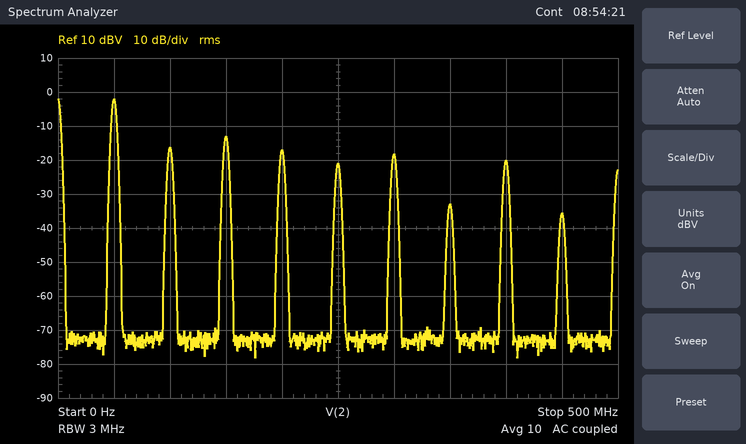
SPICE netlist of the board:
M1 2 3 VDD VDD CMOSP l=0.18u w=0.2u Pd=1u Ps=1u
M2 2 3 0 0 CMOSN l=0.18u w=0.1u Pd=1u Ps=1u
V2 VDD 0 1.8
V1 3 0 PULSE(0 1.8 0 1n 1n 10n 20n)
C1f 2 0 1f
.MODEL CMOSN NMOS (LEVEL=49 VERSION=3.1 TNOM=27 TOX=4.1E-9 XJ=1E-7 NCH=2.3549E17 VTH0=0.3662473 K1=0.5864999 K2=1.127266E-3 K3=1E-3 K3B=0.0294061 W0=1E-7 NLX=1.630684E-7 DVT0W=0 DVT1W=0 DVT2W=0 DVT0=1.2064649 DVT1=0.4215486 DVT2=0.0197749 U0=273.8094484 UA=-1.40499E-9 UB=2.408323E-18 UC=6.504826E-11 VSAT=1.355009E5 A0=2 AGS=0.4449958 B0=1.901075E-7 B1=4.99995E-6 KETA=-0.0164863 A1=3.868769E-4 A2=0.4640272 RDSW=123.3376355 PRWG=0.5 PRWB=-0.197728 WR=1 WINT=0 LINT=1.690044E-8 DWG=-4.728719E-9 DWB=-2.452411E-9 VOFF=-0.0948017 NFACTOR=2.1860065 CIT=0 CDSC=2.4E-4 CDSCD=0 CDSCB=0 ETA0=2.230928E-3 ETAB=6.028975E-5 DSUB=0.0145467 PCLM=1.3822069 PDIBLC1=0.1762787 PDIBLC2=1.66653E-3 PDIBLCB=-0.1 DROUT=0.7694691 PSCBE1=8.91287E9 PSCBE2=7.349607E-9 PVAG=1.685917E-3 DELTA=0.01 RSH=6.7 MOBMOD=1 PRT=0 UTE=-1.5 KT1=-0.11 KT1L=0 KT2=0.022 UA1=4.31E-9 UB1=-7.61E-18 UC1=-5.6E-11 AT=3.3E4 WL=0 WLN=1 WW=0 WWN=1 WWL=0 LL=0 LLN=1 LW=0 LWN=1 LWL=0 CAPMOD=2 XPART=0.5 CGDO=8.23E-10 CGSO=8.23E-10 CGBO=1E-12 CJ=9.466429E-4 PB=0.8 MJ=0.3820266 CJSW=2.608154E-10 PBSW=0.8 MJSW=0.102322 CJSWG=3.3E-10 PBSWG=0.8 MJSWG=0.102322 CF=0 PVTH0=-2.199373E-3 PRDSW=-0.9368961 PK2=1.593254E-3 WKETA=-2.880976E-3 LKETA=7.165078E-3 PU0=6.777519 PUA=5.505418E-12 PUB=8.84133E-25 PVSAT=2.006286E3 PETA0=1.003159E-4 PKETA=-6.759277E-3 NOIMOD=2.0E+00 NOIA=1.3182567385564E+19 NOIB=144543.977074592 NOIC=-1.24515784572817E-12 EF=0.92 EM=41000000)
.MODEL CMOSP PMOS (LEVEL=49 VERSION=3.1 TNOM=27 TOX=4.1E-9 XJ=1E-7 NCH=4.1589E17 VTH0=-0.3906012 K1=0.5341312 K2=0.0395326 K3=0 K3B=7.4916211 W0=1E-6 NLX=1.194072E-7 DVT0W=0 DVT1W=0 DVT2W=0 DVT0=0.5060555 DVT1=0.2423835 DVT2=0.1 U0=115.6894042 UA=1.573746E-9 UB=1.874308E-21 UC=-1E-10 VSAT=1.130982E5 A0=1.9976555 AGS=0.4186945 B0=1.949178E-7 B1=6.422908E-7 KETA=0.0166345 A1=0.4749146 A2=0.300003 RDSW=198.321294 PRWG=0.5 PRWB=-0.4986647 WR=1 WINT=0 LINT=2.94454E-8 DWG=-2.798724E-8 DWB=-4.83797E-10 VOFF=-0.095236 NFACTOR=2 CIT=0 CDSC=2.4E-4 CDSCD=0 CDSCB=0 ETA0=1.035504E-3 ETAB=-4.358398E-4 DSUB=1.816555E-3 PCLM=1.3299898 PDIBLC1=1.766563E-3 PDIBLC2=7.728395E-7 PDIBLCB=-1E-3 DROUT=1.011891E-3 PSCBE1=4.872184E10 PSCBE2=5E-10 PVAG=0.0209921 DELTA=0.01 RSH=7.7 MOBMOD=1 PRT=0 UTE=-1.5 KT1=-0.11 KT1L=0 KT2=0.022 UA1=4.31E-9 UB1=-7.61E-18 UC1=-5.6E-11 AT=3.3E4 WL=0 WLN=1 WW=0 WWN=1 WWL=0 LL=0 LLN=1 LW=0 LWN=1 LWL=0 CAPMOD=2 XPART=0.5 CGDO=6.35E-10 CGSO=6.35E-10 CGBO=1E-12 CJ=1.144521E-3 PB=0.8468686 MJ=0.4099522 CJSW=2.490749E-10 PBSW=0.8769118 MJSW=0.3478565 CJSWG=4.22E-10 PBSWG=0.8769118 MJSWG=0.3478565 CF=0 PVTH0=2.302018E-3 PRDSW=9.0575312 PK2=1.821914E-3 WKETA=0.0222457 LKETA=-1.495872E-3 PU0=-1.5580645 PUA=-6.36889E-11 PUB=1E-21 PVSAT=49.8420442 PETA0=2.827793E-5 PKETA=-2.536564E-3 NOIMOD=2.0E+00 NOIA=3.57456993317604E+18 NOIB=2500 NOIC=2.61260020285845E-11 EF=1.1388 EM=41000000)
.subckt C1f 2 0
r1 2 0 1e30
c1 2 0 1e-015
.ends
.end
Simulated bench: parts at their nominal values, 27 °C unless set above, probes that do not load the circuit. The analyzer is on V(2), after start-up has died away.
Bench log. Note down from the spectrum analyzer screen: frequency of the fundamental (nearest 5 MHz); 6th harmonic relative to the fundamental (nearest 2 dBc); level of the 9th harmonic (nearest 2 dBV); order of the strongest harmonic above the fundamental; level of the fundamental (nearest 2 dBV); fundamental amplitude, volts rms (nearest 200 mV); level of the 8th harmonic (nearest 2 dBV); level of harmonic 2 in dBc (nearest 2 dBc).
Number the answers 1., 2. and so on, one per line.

1. 50 MHz
2. -16 dBc
3. -36 dBV
4. 3
5. -2 dBV
6. 800 mV
7. -20 dBV
8. -14 dBc
